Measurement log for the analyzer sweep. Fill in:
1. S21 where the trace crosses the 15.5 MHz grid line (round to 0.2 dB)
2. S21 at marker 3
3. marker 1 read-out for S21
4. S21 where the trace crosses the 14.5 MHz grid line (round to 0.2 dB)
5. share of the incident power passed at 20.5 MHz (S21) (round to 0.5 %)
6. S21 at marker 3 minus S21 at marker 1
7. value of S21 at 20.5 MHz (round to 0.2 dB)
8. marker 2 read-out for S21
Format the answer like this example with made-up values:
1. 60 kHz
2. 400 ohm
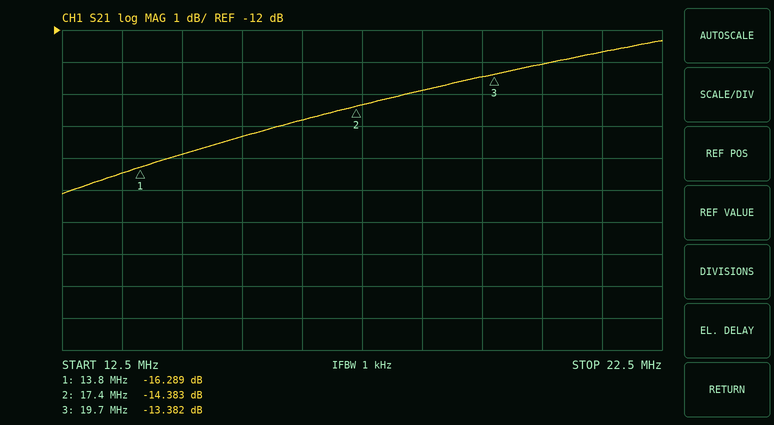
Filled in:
1. -15.4 dB
2. -13.382 dB
3. -16.289 dB
4. -15.8 dB
5. 5.0 %
6. 2.907 dB
7. -13.0 dB
8. -14.383 dB
